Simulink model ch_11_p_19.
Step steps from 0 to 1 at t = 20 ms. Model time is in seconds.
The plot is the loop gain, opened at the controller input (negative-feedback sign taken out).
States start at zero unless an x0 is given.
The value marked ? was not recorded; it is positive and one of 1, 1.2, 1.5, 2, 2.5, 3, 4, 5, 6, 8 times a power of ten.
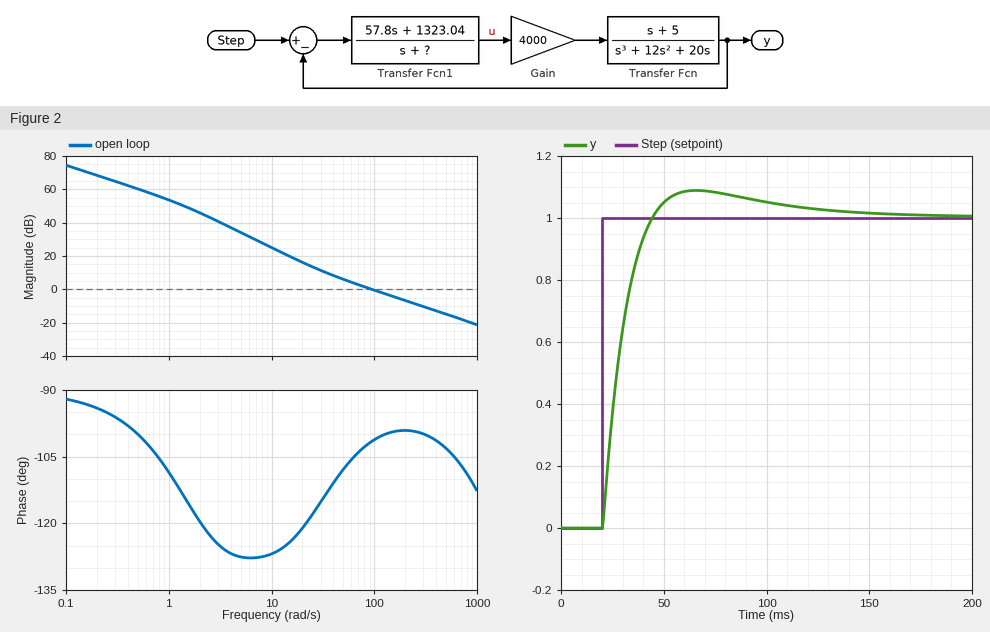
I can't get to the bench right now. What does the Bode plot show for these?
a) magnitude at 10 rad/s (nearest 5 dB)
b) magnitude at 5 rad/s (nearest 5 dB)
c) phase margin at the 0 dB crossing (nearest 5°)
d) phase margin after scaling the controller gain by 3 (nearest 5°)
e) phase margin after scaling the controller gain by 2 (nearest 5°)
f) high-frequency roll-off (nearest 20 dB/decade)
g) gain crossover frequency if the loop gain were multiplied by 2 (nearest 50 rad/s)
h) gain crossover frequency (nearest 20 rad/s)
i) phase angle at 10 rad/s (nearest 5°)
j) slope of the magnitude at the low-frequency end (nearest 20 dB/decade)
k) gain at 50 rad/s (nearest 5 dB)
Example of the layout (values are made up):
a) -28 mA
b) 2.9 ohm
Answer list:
a) 25 dB
b) 35 dB
c) 80°
d) 80°
e) 80°
f) -20 dB/decade
g) 200 rad/s
h) 100 rad/s
i) -125°
j) -20 dB/decade
k) 5 dB
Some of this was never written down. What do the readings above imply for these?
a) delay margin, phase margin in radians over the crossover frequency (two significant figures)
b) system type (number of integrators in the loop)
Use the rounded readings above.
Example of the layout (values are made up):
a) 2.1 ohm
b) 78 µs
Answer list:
a) 0.014 s
b) 1
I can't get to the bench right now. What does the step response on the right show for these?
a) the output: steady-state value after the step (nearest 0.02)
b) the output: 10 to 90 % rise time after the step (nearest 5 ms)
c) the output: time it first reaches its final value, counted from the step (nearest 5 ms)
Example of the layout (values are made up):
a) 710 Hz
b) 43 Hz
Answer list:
a) 1.00
b) 15 ms
c) 25 ms
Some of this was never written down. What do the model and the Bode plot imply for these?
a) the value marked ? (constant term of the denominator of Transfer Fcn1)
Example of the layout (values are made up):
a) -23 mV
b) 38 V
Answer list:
a) 2500
